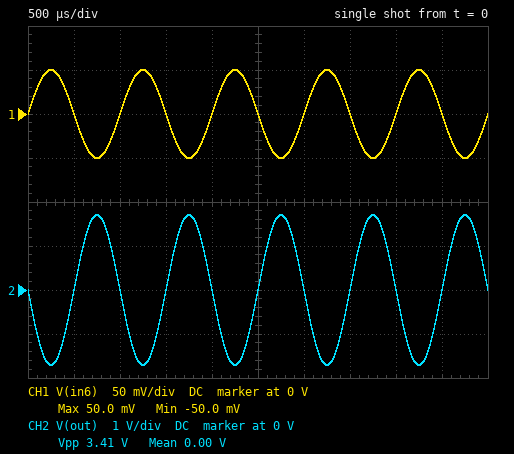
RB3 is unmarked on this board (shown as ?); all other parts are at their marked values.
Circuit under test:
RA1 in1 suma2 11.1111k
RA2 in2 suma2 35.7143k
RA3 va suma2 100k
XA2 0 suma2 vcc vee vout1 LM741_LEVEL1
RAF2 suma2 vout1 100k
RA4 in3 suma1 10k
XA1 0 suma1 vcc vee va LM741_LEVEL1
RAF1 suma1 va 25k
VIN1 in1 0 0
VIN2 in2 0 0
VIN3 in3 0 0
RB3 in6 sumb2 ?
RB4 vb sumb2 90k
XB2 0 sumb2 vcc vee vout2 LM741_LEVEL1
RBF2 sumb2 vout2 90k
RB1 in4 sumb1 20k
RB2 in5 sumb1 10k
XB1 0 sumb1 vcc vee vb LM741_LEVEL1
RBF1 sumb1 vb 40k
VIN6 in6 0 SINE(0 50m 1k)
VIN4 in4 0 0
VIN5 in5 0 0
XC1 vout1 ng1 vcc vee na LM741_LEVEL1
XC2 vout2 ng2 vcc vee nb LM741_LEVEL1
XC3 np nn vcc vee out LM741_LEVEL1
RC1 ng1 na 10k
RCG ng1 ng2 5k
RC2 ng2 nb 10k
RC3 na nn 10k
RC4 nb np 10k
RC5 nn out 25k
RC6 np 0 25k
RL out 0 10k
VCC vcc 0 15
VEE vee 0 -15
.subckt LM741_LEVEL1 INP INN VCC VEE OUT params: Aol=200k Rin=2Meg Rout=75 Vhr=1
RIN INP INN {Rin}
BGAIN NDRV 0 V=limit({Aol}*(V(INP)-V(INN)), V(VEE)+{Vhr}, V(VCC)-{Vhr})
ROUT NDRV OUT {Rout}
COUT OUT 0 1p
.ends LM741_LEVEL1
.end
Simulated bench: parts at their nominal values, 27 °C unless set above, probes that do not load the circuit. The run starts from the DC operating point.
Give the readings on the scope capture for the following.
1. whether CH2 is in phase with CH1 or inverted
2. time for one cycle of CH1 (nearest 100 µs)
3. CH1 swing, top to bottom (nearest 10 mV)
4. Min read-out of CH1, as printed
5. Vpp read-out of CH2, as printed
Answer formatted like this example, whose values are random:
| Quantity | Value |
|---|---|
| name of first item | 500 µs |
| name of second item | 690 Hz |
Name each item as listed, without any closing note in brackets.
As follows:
| Quantity | Value |
|---|---|
| whether CH2 is in phase with CH1 or inverted | inverted |
| time for one cycle of CH1 | 1.0 ms |
| CH1 swing, top to bottom | 100 mV |
| Min read-out of CH1, as printed | -50.0 mV |
| Vpp read-out of CH2, as printed | 3.41 V |
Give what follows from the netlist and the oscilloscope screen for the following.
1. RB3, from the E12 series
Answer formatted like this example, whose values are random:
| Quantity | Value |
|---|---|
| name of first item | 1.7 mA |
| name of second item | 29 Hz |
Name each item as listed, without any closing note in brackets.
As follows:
| Quantity | Value |
|---|---|
| RB3, from the E12 series | 33 kΩ |
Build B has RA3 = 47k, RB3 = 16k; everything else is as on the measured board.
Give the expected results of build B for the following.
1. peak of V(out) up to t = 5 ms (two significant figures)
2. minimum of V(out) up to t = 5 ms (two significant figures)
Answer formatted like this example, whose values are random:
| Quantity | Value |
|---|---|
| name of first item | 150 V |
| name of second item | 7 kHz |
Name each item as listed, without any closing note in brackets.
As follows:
| Quantity | Value |
|---|---|
| peak of V(out) up to t = 5 ms | 3.5 V |
| minimum of V(out) up to t = 5 ms | -3.5 V |
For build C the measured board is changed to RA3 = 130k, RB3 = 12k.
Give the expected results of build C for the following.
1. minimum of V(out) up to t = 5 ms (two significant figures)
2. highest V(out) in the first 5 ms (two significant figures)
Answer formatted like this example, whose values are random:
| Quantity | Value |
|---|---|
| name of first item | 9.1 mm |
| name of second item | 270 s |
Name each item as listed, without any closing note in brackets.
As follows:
| Quantity | Value |
|---|---|
| minimum of V(out) up to t = 5 ms | -4.7 V |
| highest V(out) in the first 5 ms | 4.7 V |
